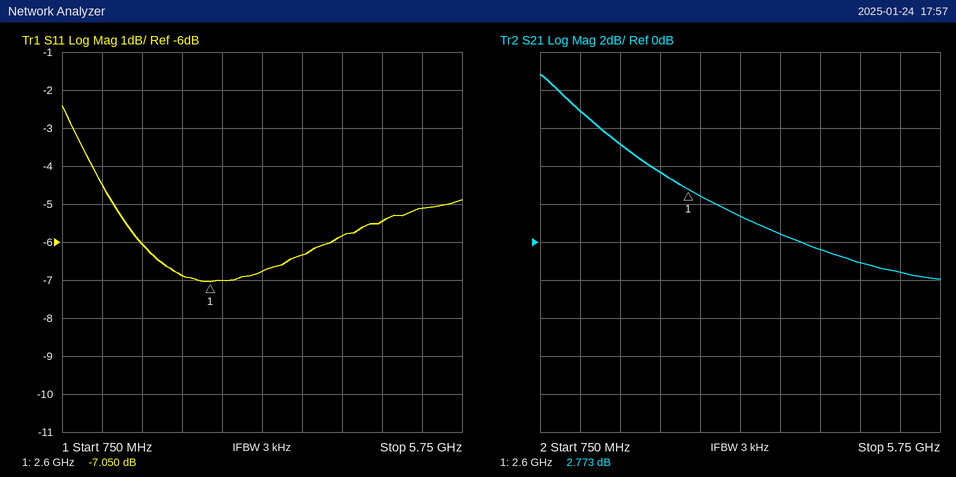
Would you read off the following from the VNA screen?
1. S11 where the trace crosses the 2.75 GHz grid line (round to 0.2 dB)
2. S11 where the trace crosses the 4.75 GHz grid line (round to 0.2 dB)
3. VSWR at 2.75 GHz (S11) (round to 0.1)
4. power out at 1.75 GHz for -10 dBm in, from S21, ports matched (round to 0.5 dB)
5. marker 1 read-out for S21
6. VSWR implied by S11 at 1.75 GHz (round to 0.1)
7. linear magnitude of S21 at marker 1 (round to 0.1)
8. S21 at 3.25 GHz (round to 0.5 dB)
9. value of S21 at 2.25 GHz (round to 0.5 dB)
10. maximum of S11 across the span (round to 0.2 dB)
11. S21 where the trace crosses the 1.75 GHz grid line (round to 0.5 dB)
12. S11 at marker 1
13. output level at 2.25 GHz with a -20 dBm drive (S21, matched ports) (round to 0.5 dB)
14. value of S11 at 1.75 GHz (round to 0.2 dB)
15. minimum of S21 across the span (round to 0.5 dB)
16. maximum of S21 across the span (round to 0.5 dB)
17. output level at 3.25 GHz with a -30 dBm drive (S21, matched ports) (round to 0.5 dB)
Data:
-7.0 dB
-5.4 dB
2.6
-5.0 dBm
2.773 dB
3.0
1.4
1.5 dB
3.5 dB
-2.4 dB
5.0 dB
-7.050 dB
-16.5 dBm
-6.0 dB
-2.0 dB
9.0 dB
-28.5 dBm
